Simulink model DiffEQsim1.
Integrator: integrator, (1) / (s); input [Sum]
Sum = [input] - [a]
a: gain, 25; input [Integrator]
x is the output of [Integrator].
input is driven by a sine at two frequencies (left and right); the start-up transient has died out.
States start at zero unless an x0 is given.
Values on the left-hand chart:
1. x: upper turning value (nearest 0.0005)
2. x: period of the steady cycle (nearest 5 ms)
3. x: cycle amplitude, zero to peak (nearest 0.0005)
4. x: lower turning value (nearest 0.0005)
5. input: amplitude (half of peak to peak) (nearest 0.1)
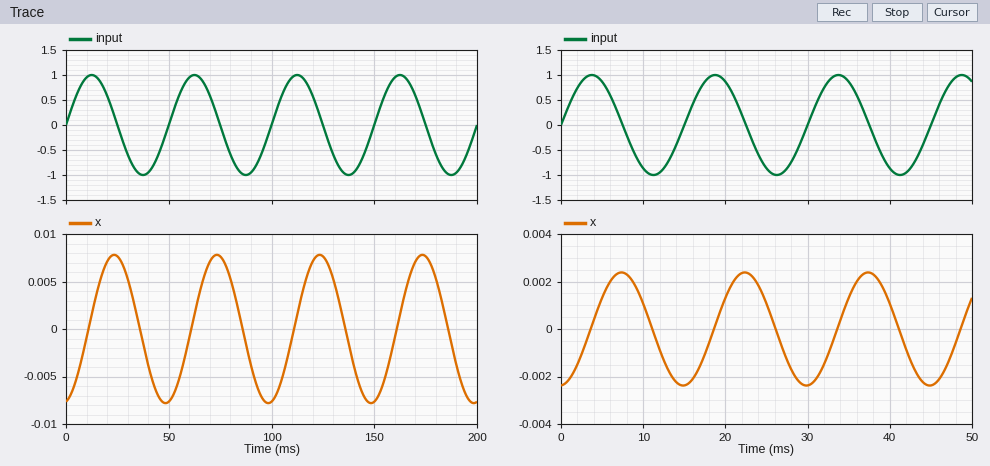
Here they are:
0.0080
50 ms
0.0080
-0.0080
1.0
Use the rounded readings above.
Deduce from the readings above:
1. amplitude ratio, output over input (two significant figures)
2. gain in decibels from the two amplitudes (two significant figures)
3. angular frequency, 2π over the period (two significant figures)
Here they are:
0.0080
-42 dB
0.13 rad/ms
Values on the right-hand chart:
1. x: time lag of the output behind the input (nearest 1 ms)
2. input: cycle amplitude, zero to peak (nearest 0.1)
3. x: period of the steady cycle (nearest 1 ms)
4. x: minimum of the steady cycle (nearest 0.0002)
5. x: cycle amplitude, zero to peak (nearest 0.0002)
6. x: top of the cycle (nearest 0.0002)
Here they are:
4 ms
1.0
15 ms
-0.0024
0.0024
0.0024
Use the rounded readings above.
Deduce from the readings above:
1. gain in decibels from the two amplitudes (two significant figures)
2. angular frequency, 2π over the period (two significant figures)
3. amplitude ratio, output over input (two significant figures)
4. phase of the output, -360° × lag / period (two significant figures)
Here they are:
-52 dB
0.42 rad/ms
0.0024
-96°
